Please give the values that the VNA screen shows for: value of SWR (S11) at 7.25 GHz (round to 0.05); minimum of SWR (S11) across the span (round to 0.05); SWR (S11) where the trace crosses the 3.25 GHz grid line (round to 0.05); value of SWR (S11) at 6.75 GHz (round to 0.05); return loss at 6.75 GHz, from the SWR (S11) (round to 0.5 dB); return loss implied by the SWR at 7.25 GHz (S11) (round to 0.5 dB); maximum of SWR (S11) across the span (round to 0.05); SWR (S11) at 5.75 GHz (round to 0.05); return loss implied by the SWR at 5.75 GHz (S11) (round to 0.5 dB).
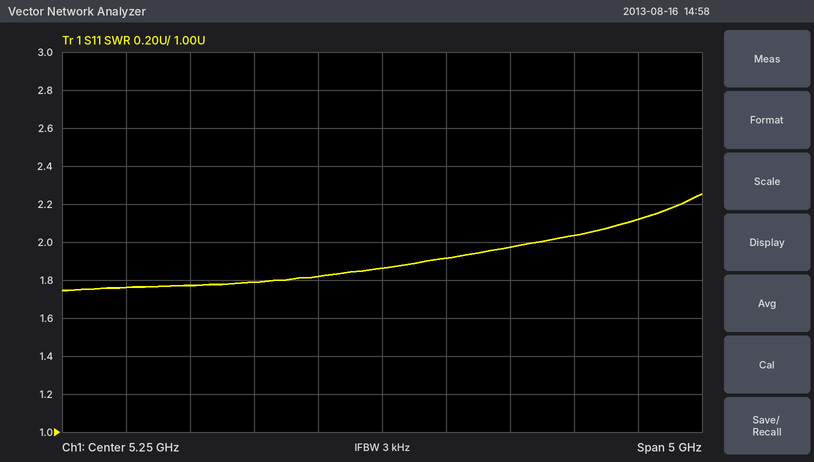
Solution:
2.10
1.75
1.75
2.05
9.5 dB
9.0 dB
2.25
1.90
10.0 dB
